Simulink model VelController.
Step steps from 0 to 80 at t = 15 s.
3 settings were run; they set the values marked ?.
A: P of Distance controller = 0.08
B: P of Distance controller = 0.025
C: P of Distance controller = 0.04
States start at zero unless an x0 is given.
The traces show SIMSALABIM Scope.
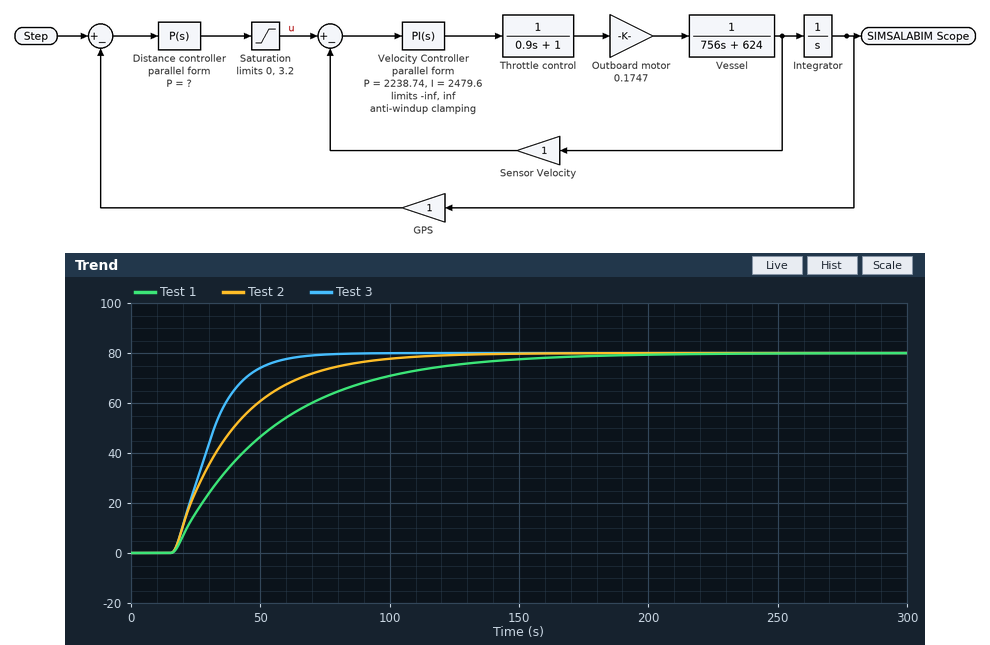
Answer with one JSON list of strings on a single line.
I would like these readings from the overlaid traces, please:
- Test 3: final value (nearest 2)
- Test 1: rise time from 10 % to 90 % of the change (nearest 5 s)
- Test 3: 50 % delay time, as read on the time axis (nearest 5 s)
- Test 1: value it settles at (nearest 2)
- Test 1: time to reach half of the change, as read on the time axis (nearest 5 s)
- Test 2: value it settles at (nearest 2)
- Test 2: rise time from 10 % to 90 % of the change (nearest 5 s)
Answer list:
["80", "85 s", "30 s", "80", "45 s", "80", "50 s"]
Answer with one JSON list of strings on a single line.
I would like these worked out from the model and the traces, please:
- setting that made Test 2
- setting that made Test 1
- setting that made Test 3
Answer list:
["C", "B", "A"]
